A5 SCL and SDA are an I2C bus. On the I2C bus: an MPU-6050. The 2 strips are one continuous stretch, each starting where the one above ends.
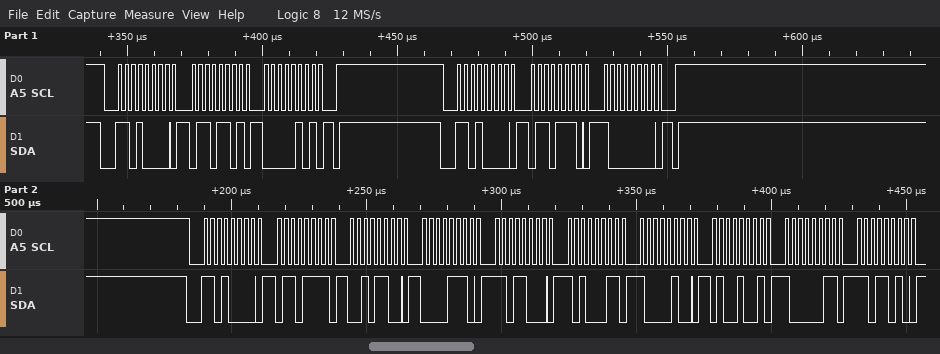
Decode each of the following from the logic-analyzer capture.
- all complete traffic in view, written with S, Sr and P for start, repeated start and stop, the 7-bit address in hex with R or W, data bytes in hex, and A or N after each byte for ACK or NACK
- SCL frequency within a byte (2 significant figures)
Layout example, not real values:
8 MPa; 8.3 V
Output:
S 68W A 6D A 05 A P S 68W A 6E A 80 A P S 68W A 6F A 2C A 0E A D8 A A3 A 84 A 49 A 83 A DA A; 400 kHz
